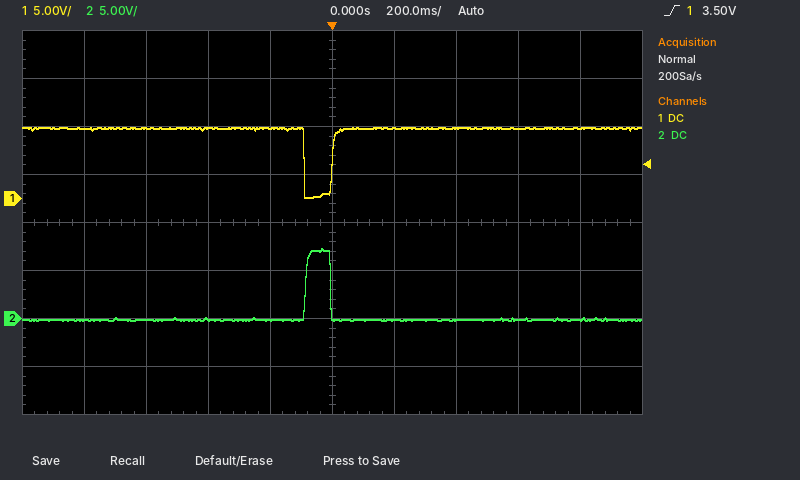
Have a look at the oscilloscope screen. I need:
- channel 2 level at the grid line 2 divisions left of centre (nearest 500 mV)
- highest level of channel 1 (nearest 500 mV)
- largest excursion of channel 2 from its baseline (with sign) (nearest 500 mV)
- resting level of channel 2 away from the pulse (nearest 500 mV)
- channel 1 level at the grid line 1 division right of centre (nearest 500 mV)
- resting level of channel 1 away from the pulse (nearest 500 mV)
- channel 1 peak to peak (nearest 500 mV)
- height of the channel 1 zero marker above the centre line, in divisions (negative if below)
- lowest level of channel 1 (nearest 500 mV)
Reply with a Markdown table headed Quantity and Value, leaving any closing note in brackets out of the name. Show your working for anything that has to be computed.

| Quantity | Value |
|---|---|
| channel 2 level at the grid line 2 divisions left of centre | 0.0 V |
| highest level of channel 1 | 7.5 V |
| largest excursion of channel 2 from its baseline (with sign) | +7.5 V |
| resting level of channel 2 away from the pulse | 0.0 V |
| channel 1 level at the grid line 1 division right of centre | 7.5 V |
| resting level of channel 1 away from the pulse | 7.5 V |
| channel 1 peak to peak | 7.5 V − (0.0 V) = 7.5 V |
| height of the channel 1 zero marker above the centre line, in divisions | +0.5 div |
| lowest level of channel 1 | 0.0 V |
